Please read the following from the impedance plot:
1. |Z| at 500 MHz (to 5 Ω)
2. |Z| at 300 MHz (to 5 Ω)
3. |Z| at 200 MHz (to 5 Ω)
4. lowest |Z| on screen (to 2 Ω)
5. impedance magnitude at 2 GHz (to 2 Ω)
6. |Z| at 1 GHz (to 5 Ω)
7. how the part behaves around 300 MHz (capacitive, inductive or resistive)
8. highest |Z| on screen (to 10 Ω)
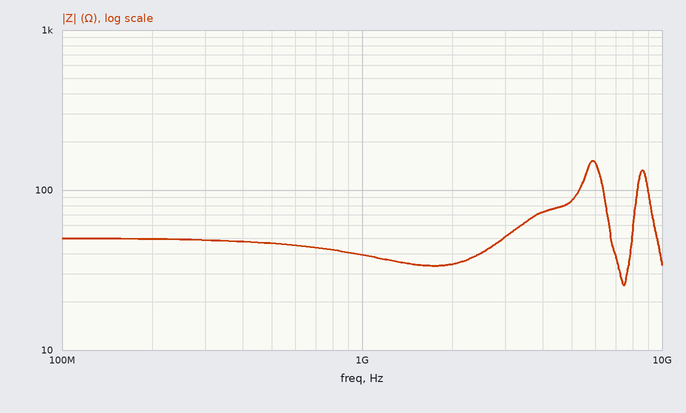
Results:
45 Ω
50 Ω
50 Ω
26 Ω
34 Ω
40 Ω
resistive
150 Ω
